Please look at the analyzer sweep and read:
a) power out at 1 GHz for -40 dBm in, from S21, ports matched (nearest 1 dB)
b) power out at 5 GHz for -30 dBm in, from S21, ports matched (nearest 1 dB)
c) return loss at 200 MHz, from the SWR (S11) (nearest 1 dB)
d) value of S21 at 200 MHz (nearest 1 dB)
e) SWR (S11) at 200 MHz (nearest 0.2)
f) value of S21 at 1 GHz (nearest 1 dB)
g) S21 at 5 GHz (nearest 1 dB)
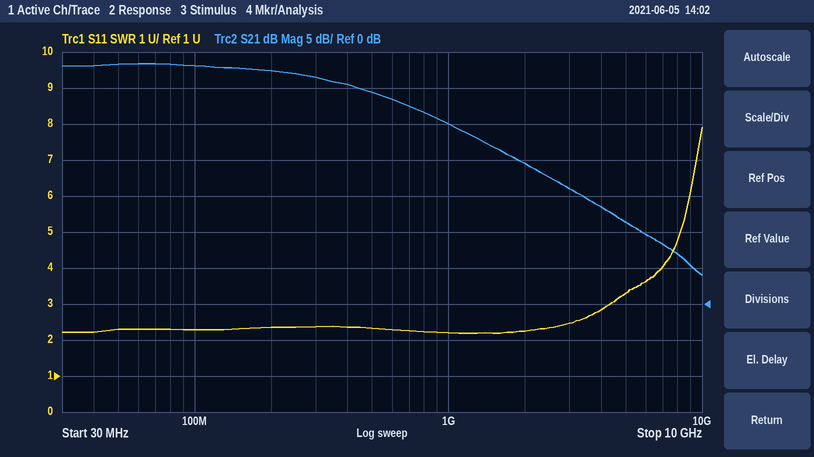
-15 dBm
-19 dBm
8 dB
32 dB
2.4
25 dB
11 dB
